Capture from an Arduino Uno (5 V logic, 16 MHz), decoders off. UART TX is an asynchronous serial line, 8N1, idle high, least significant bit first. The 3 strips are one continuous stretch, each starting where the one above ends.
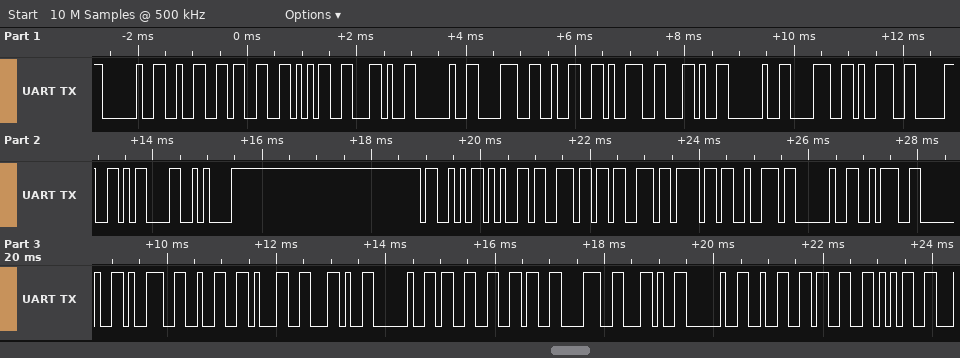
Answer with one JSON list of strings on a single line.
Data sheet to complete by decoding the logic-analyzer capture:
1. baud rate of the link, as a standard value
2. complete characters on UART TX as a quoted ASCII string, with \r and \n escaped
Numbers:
["9600 baud", "\" 235, 829, 890\\r\\nSensor : 921, 368, 235\""]
